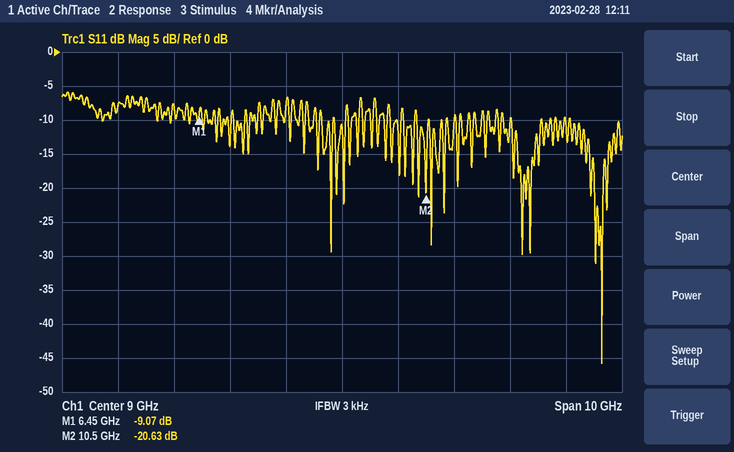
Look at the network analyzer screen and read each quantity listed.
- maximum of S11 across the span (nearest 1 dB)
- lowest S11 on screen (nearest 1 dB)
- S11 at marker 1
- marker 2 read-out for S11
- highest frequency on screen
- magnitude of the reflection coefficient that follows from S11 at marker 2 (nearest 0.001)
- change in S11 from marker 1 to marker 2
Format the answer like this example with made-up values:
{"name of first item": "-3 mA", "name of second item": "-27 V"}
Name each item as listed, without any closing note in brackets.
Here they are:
{"maximum of S11 across the span": "-6 dB", "lowest S11 on screen": "-46 dB", "S11 at marker 1": "-9.07 dB", "marker 2 read-out for S11": "-20.63 dB", "highest frequency on screen": "14 GHz", "magnitude of the reflection coefficient that follows from S11 at marker 2": "0.093", "change in S11 from marker 1 to marker 2": "-11.56 dB"}
